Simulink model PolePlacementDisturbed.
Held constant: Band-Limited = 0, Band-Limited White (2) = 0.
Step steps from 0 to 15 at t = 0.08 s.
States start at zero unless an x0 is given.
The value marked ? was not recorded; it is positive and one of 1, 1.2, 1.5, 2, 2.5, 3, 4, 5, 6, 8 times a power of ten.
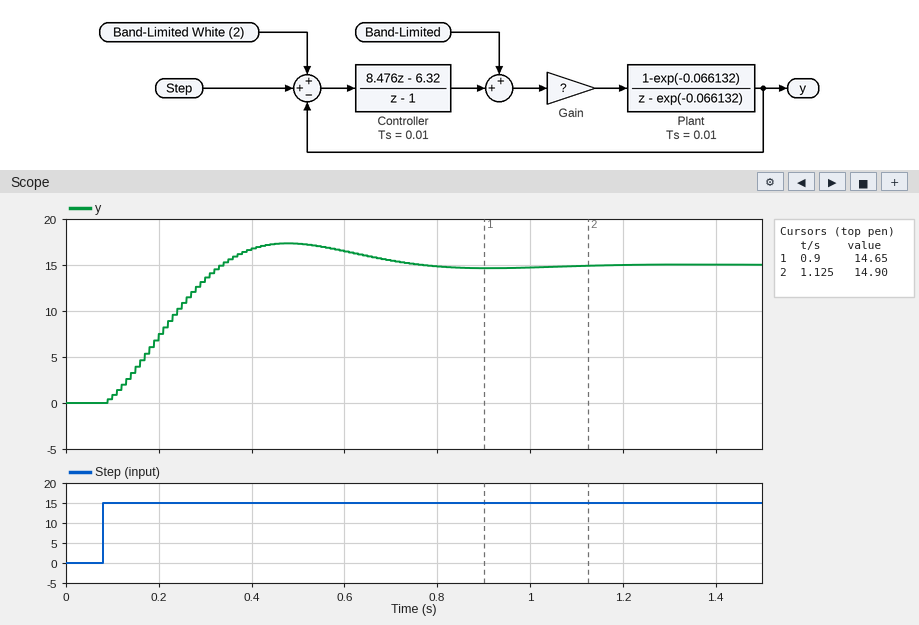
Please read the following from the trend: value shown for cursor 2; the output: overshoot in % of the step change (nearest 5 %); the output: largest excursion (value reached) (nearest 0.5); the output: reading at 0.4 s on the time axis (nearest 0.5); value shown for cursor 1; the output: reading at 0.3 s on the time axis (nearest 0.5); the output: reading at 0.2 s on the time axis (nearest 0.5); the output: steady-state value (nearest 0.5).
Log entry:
14.90
15 %
17.5
17.0
14.65
13.5
7.5
15.0
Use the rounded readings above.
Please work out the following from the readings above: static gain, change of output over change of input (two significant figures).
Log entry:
1.0
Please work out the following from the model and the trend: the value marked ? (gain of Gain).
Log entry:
0.05
